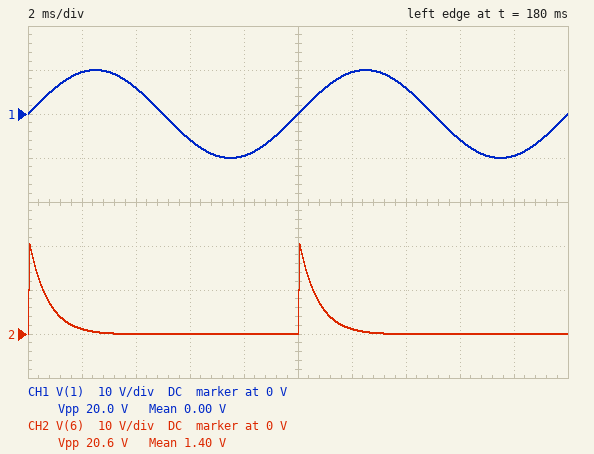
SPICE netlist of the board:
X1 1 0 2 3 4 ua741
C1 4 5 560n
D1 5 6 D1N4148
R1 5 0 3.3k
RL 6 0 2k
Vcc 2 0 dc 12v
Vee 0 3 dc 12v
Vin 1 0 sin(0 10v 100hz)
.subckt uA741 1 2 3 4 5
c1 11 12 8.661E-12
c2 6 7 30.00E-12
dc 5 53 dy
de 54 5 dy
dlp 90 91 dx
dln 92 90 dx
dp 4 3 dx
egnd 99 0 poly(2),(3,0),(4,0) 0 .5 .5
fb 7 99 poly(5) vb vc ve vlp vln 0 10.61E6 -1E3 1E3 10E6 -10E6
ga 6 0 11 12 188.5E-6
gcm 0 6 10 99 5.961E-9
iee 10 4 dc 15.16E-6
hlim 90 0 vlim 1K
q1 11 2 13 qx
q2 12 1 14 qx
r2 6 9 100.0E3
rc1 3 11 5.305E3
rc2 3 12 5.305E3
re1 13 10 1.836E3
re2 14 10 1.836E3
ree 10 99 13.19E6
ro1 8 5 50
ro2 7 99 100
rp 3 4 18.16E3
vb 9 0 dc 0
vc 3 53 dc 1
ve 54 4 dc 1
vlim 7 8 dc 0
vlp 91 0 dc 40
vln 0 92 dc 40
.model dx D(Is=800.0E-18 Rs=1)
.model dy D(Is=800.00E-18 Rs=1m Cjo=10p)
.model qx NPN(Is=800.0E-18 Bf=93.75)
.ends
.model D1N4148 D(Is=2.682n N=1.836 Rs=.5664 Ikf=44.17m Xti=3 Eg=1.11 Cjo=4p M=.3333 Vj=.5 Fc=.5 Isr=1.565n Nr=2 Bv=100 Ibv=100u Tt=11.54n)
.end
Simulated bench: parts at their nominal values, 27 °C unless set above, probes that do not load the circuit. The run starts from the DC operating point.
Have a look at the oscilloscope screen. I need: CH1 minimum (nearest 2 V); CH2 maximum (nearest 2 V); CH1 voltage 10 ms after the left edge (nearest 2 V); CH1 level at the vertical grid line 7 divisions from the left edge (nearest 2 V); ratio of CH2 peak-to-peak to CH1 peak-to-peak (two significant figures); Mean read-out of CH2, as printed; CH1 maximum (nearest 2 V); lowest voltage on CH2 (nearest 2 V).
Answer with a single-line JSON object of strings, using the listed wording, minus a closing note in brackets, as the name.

{"CH1 minimum": "-10 V", "CH2 maximum": "20 V", "CH1 voltage 10 ms after the left edge": "0 V", "CH1 level at the vertical grid line 7 divisions from the left edge": "6 V", "ratio of CH2 peak-to-peak to CH1 peak-to-peak": "1.0", "Mean read-out of CH2, as printed": "1.40 V", "CH1 maximum": "10 V", "lowest voltage on CH2": "0 V"}
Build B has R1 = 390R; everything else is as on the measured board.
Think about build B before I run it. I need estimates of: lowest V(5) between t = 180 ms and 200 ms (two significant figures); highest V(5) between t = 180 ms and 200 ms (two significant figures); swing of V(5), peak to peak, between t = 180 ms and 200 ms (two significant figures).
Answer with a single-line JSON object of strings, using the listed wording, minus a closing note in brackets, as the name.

{"lowest V(5) between t = 180 ms and 200 ms": "-16 V", "highest V(5) between t = 180 ms and 200 ms": "13 V", "swing of V(5), peak to peak, between t = 180 ms and 200 ms": "29 V"}
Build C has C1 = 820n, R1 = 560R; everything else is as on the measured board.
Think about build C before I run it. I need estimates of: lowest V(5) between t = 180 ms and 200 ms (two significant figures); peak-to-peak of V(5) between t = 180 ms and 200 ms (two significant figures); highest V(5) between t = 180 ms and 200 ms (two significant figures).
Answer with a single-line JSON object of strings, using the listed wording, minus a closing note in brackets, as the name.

{"lowest V(5) between t = 180 ms and 200 ms": "-22 V", "peak-to-peak of V(5) between t = 180 ms and 200 ms": "40 V", "highest V(5) between t = 180 ms and 200 ms": "18 V"}
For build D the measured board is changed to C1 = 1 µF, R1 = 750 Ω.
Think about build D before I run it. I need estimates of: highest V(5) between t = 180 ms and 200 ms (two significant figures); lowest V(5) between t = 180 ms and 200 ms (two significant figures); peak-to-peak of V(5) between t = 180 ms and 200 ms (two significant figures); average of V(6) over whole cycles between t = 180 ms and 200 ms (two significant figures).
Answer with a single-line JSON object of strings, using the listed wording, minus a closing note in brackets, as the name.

{"highest V(5) between t = 180 ms and 200 ms": "22 V", "lowest V(5) between t = 180 ms and 200 ms": "-23 V", "peak-to-peak of V(5) between t = 180 ms and 200 ms": "45 V", "average of V(6) over whole cycles between t = 180 ms and 200 ms": "1.2 V"}
